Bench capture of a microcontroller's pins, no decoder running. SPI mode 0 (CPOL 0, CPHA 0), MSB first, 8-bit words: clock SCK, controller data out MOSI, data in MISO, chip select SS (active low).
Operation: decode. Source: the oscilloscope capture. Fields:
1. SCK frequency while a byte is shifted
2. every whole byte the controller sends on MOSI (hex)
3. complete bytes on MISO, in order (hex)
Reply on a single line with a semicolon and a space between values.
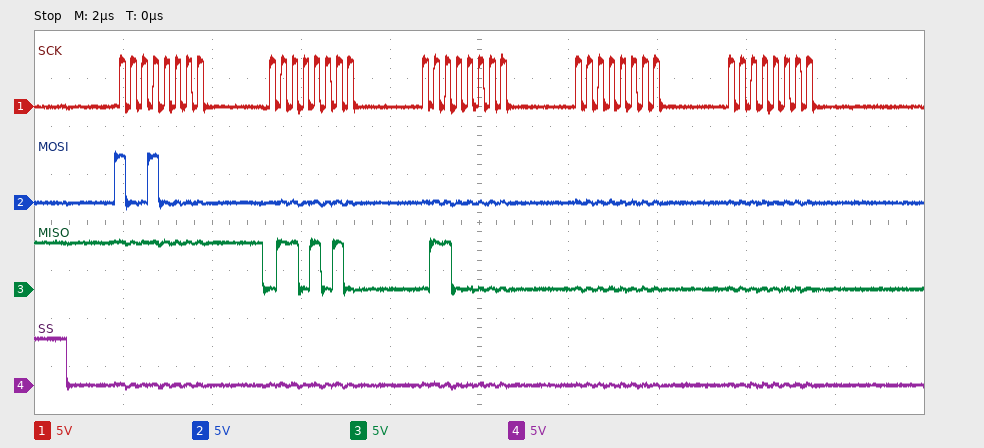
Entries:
4 MHz; 90 00 00 00 00; FF 6A 60 00 00
